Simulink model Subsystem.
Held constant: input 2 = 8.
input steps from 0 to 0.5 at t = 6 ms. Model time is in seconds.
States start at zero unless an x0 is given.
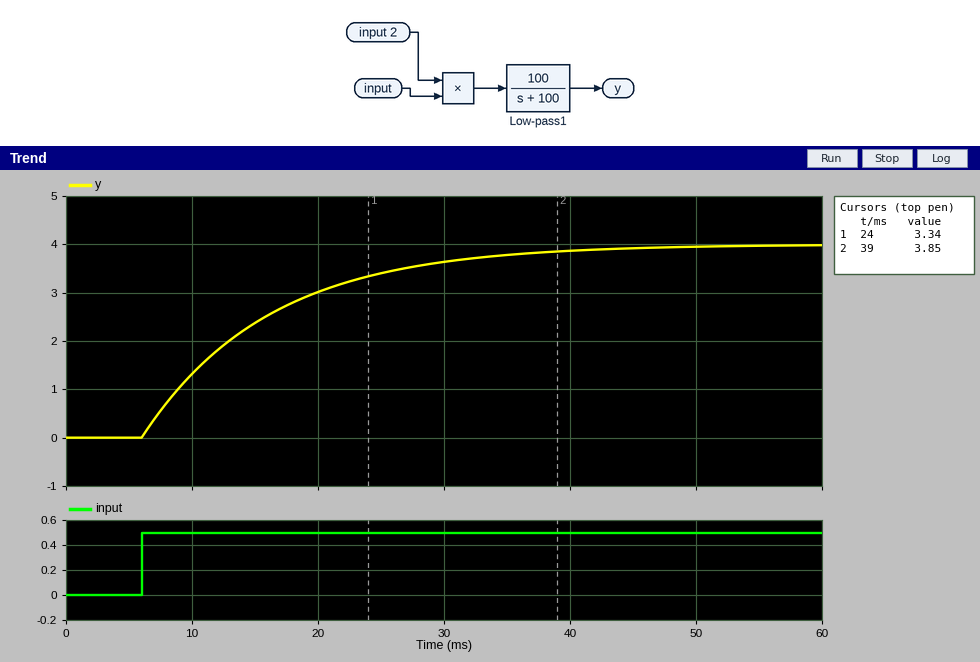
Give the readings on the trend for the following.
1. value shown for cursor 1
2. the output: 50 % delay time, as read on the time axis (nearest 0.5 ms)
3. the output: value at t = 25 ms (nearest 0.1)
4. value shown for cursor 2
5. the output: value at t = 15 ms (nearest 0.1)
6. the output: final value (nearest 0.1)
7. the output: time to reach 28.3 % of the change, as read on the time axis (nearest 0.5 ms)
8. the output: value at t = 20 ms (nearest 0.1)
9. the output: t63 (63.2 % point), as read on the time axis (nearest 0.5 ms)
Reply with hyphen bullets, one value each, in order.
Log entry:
- 3.34
- 13.0 ms
- 3.4
- 3.85
- 2.4
- 4.0
- 9.5 ms
- 3.0
- 16.0 ms
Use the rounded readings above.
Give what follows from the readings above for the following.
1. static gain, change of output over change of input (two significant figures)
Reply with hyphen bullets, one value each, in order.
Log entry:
- 8.0
